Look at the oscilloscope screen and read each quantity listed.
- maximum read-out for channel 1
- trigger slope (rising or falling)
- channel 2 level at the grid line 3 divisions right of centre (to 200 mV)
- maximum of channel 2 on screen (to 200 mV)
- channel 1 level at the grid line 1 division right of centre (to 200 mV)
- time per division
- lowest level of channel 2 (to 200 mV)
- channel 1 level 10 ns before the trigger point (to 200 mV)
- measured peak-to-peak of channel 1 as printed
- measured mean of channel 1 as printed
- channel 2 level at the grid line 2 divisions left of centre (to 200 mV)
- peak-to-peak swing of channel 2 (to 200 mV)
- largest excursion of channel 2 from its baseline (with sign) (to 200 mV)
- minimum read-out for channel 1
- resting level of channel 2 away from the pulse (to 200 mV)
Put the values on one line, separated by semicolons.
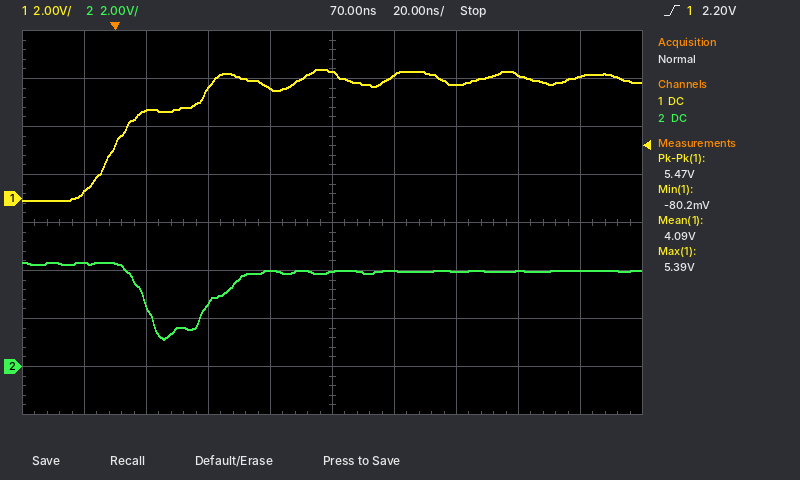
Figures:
5.39 V; rising; 4.0 V; 4.4 V; 5.2 V; 20 ns; 1.2 V; 200 mV; 5.47 V; 4.09 V; 2.6 V; 3.2 V; -2.8 V; -80.2 mV; 4.0 V
